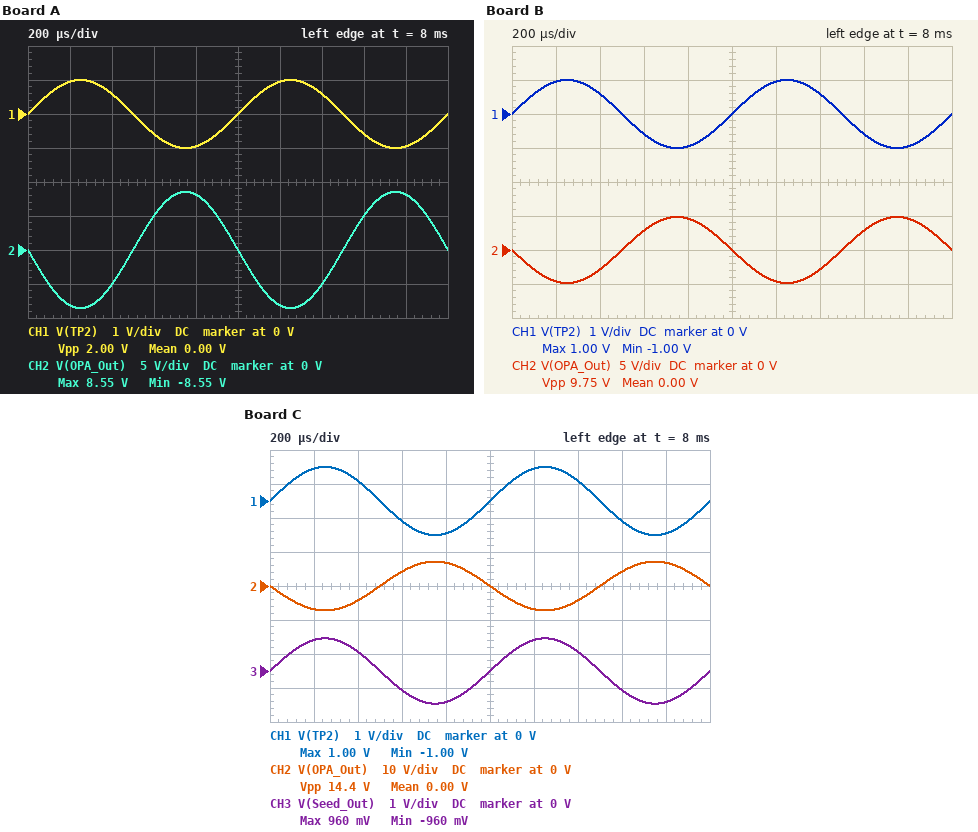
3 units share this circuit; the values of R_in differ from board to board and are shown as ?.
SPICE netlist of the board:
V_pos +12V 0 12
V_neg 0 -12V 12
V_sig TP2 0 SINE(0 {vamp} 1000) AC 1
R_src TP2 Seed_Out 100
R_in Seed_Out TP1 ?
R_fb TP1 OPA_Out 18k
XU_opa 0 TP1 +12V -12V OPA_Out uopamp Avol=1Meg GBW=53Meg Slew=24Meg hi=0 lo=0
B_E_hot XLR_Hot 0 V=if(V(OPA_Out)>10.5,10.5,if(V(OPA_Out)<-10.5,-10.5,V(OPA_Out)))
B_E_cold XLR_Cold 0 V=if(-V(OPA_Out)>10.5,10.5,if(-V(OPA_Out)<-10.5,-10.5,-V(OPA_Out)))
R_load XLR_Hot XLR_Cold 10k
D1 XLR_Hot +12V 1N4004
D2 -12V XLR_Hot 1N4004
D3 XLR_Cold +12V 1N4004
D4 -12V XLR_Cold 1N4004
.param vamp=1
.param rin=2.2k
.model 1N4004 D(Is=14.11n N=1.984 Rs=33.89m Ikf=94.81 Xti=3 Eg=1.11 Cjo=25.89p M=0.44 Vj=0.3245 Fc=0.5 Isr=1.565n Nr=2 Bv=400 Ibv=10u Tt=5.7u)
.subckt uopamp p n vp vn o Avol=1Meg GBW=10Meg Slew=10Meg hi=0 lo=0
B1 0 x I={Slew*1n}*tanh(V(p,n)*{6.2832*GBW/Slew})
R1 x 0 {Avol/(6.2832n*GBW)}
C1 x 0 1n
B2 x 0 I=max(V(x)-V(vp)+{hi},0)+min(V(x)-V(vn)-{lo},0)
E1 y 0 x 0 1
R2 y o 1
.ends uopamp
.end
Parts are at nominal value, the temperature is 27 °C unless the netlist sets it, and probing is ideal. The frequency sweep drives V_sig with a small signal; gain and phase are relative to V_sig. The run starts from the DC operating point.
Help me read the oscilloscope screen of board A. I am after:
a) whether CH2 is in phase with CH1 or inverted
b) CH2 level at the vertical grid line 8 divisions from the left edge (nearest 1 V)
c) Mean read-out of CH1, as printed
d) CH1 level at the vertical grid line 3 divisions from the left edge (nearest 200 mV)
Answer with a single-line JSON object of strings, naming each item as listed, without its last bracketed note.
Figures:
{"whether CH2 is in phase with CH1 or inverted": "inverted", "CH2 level at the vertical grid line 8 divisions from the left edge": "5 V", "Mean read-out of CH1, as printed": "0.00 V", "CH1 level at the vertical grid line 3 divisions from the left edge": "-600 mV"}
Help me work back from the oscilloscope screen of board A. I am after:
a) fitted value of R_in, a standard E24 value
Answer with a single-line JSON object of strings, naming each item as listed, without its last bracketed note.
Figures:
{"fitted value of R_in, a standard E24 value": "2 kΩ"}
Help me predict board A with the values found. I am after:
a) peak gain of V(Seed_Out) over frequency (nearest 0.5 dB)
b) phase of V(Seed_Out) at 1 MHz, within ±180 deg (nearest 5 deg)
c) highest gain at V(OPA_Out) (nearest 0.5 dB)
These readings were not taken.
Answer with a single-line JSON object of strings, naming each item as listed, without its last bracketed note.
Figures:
{"peak gain of V(Seed_Out) over frequency": "0 dB", "phase of V(Seed_Out) at 1 MHz, within ±180 deg": "0 deg", "highest gain at V(OPA_Out)": "18.5 dB"}
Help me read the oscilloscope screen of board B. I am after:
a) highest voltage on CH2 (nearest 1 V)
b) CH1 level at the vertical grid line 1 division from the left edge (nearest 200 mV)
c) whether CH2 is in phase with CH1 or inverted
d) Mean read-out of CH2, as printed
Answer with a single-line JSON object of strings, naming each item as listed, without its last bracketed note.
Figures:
{"highest voltage on CH2": "5 V", "CH1 level at the vertical grid line 1 division from the left edge": "1.0 V", "whether CH2 is in phase with CH1 or inverted": "inverted", "Mean read-out of CH2, as printed": "0.00 V"}
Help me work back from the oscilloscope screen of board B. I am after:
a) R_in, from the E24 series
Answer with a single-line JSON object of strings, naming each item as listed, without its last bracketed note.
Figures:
{"R_in, from the E24 series": "3.6 kΩ"}
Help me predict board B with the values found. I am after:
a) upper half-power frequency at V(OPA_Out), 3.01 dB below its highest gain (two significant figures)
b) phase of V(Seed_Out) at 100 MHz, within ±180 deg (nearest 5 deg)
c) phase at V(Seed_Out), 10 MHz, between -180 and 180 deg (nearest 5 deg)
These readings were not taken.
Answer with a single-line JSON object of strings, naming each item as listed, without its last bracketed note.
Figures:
{"upper half-power frequency at V(OPA_Out), 3.01 dB below its highest gain": "9.0 MHz", "phase of V(Seed_Out) at 100 MHz, within ±180 deg": "0 deg", "phase at V(Seed_Out), 10 MHz, between -180 and 180 deg": "0 deg"}
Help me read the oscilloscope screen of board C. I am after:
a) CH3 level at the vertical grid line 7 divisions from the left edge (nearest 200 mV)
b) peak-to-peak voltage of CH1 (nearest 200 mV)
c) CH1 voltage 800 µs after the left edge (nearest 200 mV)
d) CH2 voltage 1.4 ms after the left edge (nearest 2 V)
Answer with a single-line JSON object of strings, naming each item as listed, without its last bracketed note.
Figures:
{"CH3 level at the vertical grid line 7 divisions from the left edge": "600 mV", "peak-to-peak voltage of CH1": "2.0 V", "CH1 voltage 800 µs after the left edge": "-1.0 V", "CH2 voltage 1.4 ms after the left edge": "-4 V"}
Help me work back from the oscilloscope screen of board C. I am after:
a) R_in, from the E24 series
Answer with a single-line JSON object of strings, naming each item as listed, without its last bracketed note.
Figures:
{"R_in, from the E24 series": "2.4 kΩ"}
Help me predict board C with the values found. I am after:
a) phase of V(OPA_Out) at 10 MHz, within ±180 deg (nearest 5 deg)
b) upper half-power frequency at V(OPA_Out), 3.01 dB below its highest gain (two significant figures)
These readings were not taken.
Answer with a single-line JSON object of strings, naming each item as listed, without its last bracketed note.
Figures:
{"phase of V(OPA_Out) at 10 MHz, within ±180 deg": "125 deg", "upper half-power frequency at V(OPA_Out), 3.01 dB below its highest gain": "6.5 MHz"}
